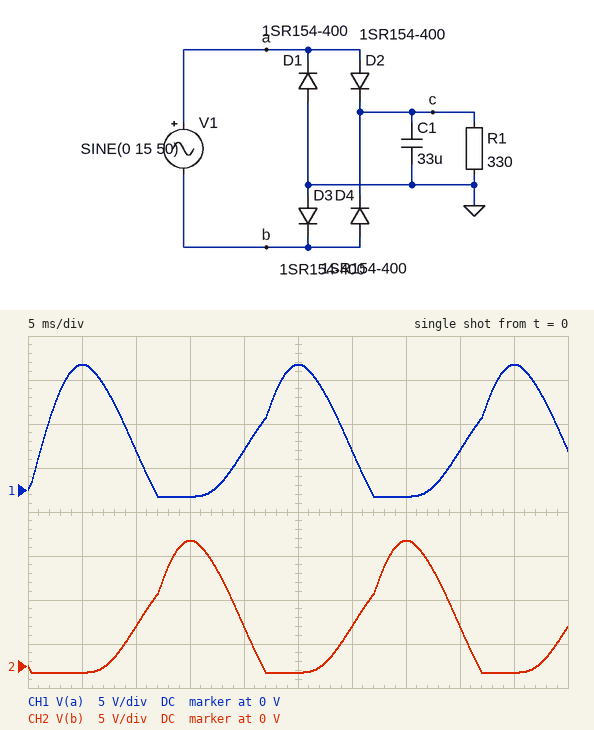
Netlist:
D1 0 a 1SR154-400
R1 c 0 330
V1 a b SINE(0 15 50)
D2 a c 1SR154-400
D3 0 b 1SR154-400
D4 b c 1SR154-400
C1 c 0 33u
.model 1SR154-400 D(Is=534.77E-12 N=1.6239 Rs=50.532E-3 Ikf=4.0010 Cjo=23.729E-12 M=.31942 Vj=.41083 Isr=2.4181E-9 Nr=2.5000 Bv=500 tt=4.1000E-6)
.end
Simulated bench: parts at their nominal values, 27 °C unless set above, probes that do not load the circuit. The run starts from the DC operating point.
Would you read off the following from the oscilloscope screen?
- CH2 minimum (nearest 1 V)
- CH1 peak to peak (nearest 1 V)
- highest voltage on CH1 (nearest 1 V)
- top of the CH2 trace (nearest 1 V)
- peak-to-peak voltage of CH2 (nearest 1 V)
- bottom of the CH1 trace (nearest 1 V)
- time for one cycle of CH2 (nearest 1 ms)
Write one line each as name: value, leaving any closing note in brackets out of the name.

CH2 minimum: -1 V
CH1 peak to peak: 15 V
highest voltage on CH1: 14 V
top of the CH2 trace: 14 V
peak-to-peak voltage of CH2: 15 V
bottom of the CH1 trace: -1 V
time for one cycle of CH2: 20 ms
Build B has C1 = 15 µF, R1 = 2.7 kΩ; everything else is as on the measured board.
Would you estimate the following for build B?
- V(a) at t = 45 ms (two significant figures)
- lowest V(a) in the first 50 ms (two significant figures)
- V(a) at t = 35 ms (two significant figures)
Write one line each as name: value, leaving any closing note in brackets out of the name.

V(a) at t = 45 ms: 14 V
lowest V(a) in the first 50 ms: -770 mV
V(a) at t = 35 ms: -700 mV
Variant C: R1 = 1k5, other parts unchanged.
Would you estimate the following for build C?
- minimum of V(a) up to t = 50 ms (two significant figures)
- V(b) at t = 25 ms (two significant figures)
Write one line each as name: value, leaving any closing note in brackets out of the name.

minimum of V(a) up to t = 50 ms: -800 mV
V(b) at t = 25 ms: -730 mV
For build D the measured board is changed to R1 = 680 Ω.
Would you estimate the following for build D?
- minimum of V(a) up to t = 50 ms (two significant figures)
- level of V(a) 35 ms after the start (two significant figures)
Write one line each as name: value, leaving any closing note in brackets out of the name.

minimum of V(a) up to t = 50 ms: -820 mV
level of V(a) 35 ms after the start: -750 mV
